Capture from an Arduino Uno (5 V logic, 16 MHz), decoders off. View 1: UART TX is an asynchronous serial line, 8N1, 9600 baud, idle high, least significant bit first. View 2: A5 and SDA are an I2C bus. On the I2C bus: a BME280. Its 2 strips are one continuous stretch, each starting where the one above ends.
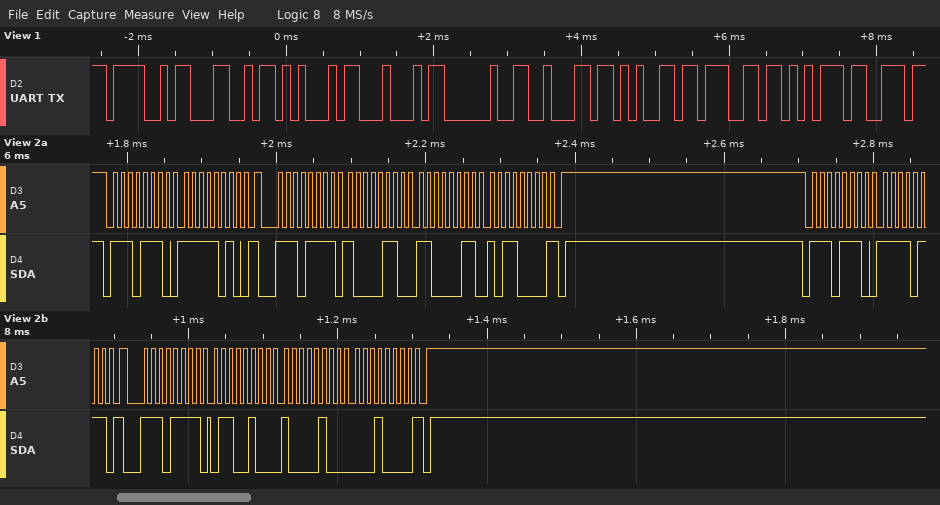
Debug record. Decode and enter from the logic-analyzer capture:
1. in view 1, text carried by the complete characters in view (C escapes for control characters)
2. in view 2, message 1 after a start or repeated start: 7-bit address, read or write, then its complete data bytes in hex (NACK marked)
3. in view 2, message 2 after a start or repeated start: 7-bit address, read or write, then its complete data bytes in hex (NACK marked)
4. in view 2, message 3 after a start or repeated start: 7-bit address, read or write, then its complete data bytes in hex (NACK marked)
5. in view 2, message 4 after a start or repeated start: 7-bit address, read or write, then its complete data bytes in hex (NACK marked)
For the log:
"OLED begu"
0x77 write: FA
0x77 read: 86 C3 B0 NACK
0x77 write: F7
0x77 read: 64 84 10 NACK
